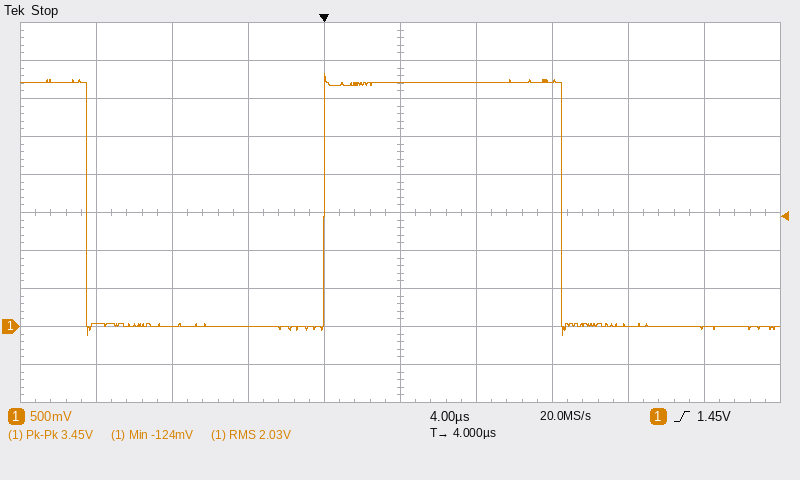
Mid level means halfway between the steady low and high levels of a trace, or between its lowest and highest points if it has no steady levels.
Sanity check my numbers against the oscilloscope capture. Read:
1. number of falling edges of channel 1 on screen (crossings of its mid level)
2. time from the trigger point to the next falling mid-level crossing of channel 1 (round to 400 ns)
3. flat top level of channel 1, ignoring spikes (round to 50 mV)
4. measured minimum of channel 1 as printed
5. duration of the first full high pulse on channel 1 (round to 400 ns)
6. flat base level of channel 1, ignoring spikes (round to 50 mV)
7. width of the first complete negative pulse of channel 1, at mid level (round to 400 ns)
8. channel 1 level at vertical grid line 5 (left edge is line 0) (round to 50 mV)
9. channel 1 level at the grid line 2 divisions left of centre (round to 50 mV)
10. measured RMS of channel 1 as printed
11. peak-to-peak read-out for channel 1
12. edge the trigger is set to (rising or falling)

2
12.4 µs
3.20 V
-124 mV
12.4 µs
0 mV
12.4 µs
3.20 V
0 mV
2.03 V
3.45 V
rising
